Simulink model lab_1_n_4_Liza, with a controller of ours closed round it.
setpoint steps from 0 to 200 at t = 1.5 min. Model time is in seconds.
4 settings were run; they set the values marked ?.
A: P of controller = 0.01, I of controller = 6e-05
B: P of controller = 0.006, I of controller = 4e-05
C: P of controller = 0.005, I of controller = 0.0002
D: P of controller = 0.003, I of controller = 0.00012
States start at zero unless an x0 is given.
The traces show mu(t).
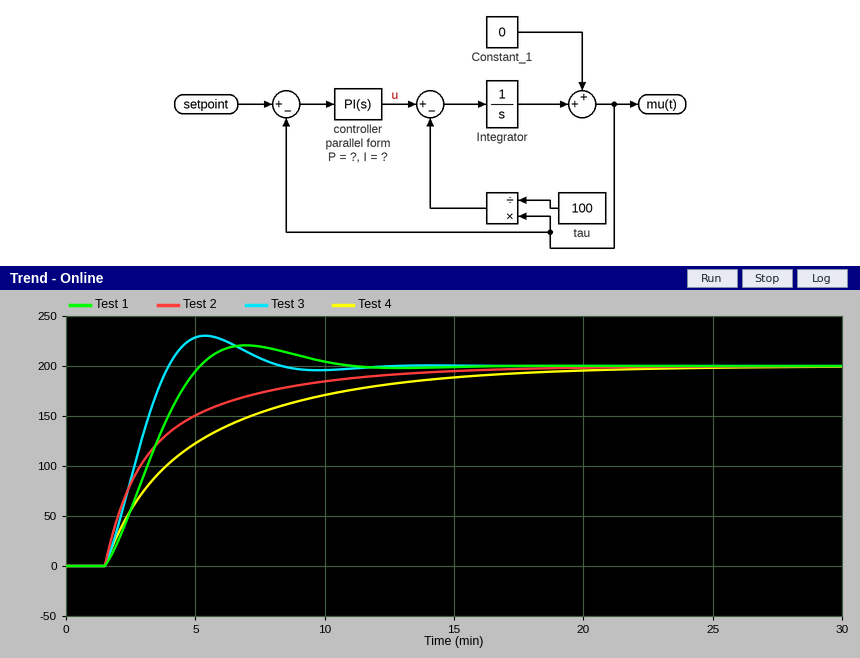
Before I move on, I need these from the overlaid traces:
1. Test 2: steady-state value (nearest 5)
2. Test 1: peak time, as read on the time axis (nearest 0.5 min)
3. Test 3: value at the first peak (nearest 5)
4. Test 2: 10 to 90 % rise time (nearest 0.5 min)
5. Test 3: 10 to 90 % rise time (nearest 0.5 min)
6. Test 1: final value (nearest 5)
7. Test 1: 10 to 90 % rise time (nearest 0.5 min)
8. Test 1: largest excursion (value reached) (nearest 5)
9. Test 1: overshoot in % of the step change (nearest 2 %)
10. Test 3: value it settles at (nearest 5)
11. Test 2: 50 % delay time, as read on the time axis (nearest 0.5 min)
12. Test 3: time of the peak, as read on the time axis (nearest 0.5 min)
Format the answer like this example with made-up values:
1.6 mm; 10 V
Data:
200; 7.0 min; 230; 7.0 min; 2.0 min; 200; 2.5 min; 220; 10 %; 200; 3.0 min; 5.5 min
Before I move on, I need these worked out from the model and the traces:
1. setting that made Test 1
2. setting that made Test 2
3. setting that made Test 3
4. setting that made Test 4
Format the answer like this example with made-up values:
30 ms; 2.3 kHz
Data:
D; A; C; B
